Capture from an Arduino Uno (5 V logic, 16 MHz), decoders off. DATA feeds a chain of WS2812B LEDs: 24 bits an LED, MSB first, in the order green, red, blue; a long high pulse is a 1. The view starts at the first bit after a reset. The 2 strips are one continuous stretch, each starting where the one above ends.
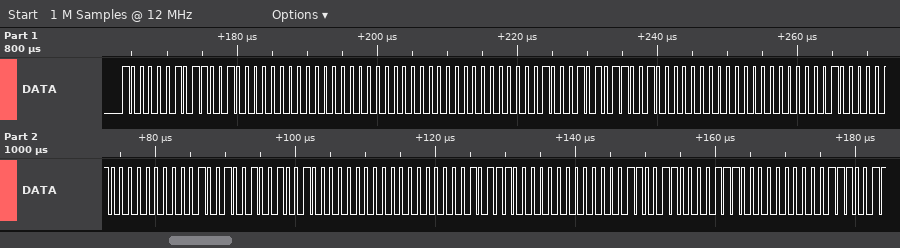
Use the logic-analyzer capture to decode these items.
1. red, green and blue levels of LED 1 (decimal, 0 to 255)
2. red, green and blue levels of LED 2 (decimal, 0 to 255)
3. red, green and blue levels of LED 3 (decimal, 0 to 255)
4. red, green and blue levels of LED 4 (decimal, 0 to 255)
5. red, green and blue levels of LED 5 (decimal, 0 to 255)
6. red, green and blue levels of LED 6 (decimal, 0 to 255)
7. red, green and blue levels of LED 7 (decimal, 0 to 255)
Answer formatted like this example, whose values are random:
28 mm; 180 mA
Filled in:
200, 130, 0; 0, 0, 0; 200, 138, 0; 65, 0, 0; 146, 36, 0; 92, 0, 0; 135, 25, 0
